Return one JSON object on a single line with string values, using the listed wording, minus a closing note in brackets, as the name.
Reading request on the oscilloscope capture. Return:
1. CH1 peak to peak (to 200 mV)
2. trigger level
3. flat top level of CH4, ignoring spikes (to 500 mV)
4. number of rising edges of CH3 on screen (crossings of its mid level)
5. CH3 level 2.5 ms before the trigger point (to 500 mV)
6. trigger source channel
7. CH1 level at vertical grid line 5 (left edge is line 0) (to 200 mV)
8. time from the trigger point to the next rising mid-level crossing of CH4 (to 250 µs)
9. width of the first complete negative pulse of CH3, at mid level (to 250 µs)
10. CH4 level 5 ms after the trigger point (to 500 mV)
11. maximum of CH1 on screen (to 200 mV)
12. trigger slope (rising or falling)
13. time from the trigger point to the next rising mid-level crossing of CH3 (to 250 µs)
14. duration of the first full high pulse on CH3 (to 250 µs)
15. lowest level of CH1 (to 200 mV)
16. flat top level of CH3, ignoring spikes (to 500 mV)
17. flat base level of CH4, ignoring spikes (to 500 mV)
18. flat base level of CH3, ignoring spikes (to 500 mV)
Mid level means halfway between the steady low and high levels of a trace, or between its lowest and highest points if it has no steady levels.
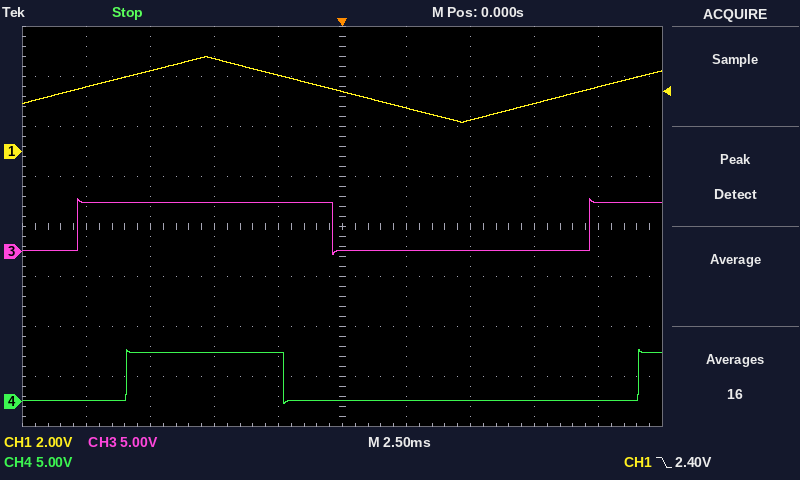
{"CH1 peak to peak": "2.6 V", "trigger level": "2.40 V", "flat top level of CH4, ignoring spikes": "5.0 V", "number of rising edges of CH3 on screen": "2", "CH3 level 2.5 ms before the trigger point": "5.0 V", "trigger source channel": "CH1", "CH1 level at vertical grid line 5 (left edge is line 0)": "2.4 V", "time from the trigger point to the next rising mid-level crossing of CH4": "11.50 ms", "width of the first complete negative pulse of CH3, at mid level": "10.00 ms", "CH4 level 5 ms after the trigger point": "0.0 V", "maximum of CH1 on screen": "3.8 V", "trigger slope": "falling", "time from the trigger point to the next rising mid-level crossing of CH3": "9.75 ms", "duration of the first full high pulse on CH3": "10.00 ms", "lowest level of CH1": "1.2 V", "flat top level of CH3, ignoring spikes": "5.0 V", "flat base level of CH4, ignoring spikes": "0.0 V", "flat base level of CH3, ignoring spikes": "0.0 V"}
